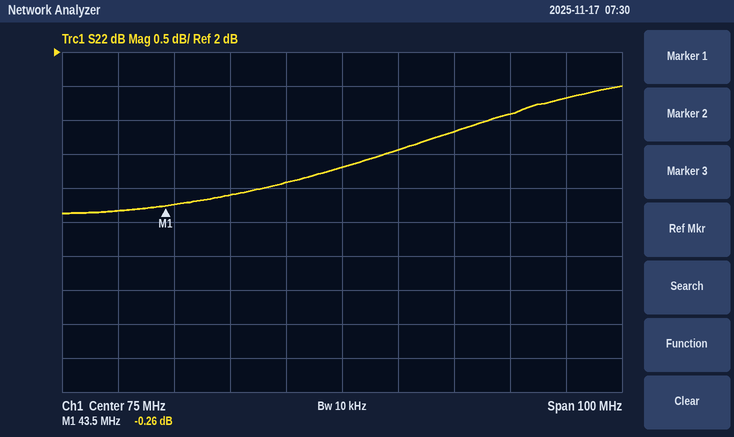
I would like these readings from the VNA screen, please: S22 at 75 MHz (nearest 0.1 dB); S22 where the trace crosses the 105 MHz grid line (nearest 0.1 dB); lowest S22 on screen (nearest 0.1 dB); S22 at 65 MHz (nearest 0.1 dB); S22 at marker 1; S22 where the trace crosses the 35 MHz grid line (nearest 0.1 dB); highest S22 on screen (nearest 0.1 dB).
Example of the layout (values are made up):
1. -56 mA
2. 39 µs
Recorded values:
1. 0.3 dB
2. 1.1 dB
3. -0.4 dB
4. 0.1 dB
5. -0.26 dB
6. -0.3 dB
7. 1.5 dB
